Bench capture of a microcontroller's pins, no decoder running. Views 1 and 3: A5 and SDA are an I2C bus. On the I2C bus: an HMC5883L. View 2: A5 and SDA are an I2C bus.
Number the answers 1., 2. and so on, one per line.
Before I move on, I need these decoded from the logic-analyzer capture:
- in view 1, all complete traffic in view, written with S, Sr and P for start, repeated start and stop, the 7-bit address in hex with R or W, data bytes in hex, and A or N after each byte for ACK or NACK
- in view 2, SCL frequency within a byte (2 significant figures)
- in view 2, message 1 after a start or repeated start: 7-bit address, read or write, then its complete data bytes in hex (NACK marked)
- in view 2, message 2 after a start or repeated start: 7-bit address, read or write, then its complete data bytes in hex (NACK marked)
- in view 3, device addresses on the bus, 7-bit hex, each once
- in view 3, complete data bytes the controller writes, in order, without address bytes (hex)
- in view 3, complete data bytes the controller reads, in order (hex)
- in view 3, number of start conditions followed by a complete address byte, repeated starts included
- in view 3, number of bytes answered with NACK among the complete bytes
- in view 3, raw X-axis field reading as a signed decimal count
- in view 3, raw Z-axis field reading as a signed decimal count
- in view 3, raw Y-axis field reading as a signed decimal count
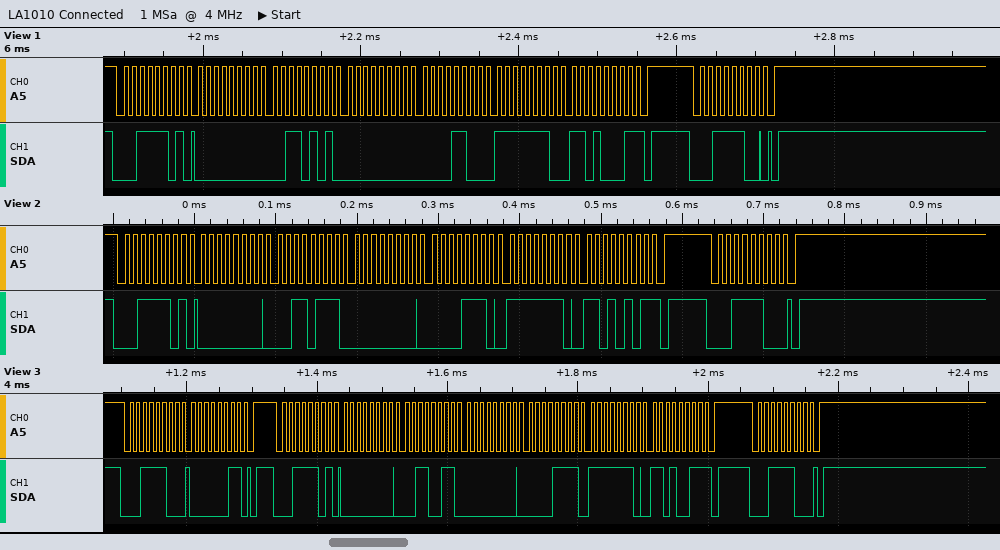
1. S 1ER A 00 A 35 A 00 A 0C A FE A D1 N P S 1EW A P
2. 100 kHz
3. 0x1E read: 00 37 00 0E FE D5 NACK
4. 0x1E write
5. 0x1E
6. 03
7. 00 33 00 0F FE D3
8. 3
9. 1
10. 51
11. 15
12. -301
